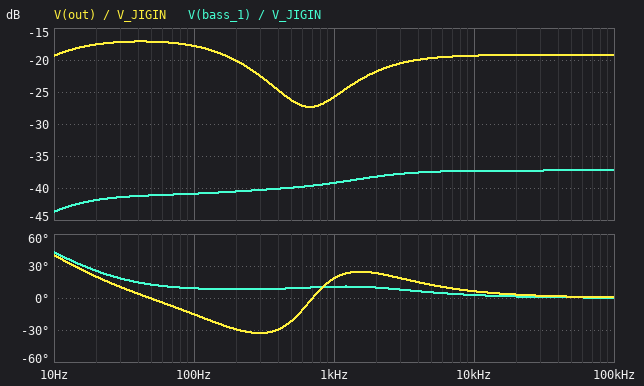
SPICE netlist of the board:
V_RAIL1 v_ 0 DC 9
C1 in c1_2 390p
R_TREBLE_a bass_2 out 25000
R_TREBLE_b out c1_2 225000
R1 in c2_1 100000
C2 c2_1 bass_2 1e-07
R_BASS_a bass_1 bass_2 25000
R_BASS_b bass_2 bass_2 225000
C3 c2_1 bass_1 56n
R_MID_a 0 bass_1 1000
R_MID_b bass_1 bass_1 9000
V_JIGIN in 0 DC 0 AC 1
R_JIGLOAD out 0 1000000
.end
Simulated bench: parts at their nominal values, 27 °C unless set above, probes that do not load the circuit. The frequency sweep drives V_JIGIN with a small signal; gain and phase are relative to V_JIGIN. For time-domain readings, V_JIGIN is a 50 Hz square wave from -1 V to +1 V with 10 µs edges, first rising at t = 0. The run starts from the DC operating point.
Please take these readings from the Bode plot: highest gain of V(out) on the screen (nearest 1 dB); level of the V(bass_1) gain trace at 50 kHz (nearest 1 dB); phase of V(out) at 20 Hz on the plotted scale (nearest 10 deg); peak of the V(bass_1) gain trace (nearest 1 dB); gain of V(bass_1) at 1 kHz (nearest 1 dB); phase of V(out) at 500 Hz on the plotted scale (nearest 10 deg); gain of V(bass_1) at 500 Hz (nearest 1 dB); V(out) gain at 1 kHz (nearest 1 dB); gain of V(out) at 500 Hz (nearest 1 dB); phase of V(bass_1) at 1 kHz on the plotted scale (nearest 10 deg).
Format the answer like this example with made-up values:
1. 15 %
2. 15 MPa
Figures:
1. -17 dB
2. -37 dB
3. 20 deg
4. -37 dB
5. -39 dB
6. -20 deg
7. -40 dB
8. -26 dB
9. -26 dB
10. 10 deg
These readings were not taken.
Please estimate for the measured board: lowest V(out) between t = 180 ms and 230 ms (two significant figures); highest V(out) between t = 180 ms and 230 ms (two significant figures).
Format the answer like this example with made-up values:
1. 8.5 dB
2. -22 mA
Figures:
1. -160 mV
2. 160 mV
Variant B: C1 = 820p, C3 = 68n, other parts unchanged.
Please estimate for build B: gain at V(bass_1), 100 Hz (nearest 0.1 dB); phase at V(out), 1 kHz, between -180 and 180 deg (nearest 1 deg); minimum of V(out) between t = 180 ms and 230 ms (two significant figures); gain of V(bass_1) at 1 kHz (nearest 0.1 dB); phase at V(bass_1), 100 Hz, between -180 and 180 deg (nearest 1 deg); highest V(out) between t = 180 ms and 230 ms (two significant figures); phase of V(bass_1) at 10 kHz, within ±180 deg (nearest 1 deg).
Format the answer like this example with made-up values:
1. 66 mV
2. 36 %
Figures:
1. -40.7 dB
2. 14 deg
3. -150 mV
4. -38.2 dB
5. 10 deg
6. 150 mV
7. 1 deg
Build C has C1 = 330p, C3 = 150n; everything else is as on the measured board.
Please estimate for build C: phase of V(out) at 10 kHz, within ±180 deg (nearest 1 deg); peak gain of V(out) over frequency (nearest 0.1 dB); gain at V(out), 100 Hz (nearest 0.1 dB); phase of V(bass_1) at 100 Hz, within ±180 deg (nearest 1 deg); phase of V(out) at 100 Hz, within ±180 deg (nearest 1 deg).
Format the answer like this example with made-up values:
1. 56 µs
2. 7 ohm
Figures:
1. 9 deg
2. -19.2 dB
3. -22.7 dB
4. 6 deg
5. -27 deg
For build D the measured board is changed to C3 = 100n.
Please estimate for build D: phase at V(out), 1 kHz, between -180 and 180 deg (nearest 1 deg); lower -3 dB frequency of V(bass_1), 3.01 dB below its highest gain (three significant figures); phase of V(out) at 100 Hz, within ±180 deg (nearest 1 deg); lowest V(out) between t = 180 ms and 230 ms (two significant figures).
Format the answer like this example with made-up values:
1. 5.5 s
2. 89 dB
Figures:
1. 32 deg
2. 195 Hz
3. -23 deg
4. -120 mV
